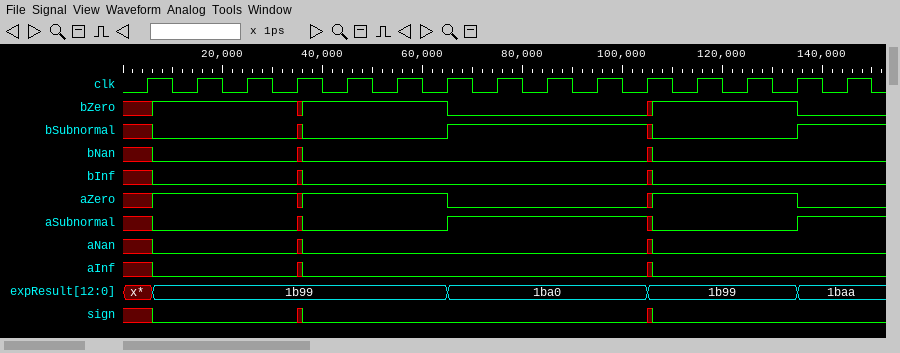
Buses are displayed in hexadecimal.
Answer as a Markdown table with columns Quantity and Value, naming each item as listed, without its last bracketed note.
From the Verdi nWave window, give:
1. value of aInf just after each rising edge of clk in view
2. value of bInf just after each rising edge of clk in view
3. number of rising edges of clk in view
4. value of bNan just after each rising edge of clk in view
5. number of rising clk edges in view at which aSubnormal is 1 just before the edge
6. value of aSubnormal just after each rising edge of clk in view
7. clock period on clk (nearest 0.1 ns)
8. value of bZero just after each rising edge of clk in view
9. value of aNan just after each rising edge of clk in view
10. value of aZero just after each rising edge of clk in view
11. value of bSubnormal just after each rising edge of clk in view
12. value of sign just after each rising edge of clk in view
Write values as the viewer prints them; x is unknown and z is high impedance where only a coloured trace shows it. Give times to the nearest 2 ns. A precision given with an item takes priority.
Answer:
| Quantity | Value |
|---|---|
| value of aInf just after each rising edge of clk in view | x 0 0 x 0 0 0 0 0 0 x 0 0 0 0 |
| value of bInf just after each rising edge of clk in view | x 0 0 x 0 0 0 0 0 0 x 0 0 0 0 |
| number of rising edges of clk in view | 15 |
| value of bNan just after each rising edge of clk in view | x 0 0 x 0 0 0 0 0 0 x 0 0 0 0 |
| number of rising clk edges in view at which aSubnormal is 1 just before the edge | 5 |
| value of aSubnormal just after each rising edge of clk in view | x 0 0 x 0 0 1 1 1 1 x 0 0 1 1 |
| clock period on clk | 10 ns |
| value of bZero just after each rising edge of clk in view | x 1 1 x 1 1 0 0 0 0 x 1 1 0 0 |
| value of aNan just after each rising edge of clk in view | x 0 0 x 0 0 0 0 0 0 x 0 0 0 0 |
| value of aZero just after each rising edge of clk in view | x 1 1 x 1 1 0 0 0 0 x 1 1 0 0 |
| value of bSubnormal just after each rising edge of clk in view | x 0 0 x 0 0 1 1 1 1 x 0 0 1 1 |
| value of sign just after each rising edge of clk in view | x 0 0 x 0 0 0 0 0 0 x 0 0 0 0 |
